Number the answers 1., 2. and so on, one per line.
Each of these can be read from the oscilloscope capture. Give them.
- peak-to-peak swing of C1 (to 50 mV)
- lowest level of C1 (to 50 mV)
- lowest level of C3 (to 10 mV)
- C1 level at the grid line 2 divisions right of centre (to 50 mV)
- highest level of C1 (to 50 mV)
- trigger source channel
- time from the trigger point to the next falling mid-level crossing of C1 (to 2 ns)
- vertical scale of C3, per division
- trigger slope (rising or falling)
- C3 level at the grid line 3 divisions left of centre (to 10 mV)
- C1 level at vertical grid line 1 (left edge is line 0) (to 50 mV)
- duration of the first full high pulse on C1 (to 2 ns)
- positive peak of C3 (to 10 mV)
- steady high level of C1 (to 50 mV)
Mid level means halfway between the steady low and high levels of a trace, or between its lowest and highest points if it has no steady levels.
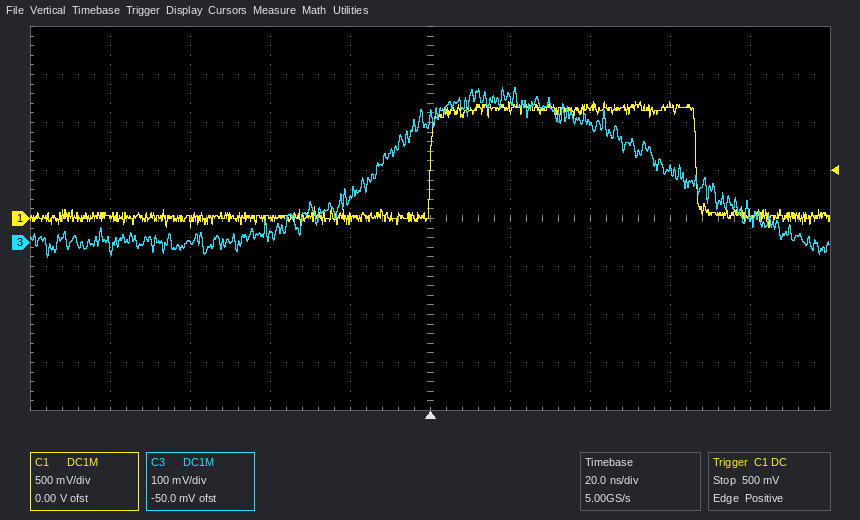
1. 1.30 V
2. -100 mV
3. -30 mV
4. 1.15 V
5. 1.20 V
6. C1
7. 66 ns
8. 100 mV
9. rising
10. 0 mV
11. 0 mV
12. 66 ns
13. 320 mV
14. 1.15 V
